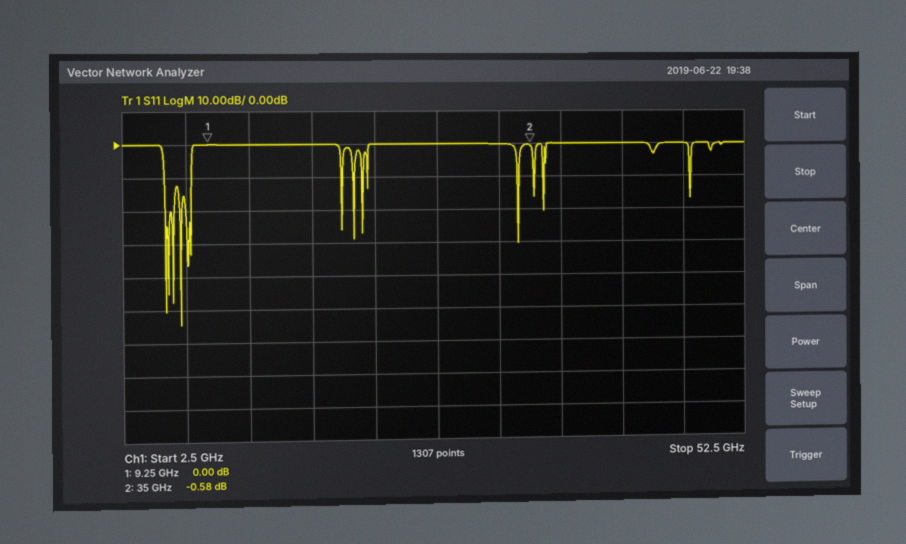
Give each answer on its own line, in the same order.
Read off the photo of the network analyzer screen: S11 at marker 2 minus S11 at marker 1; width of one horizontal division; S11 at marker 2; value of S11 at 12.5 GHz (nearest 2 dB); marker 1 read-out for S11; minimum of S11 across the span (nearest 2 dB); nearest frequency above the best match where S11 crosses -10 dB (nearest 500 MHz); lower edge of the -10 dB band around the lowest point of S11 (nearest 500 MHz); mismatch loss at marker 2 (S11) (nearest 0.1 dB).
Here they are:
-0.58 dB
5 GHz
-0.58 dB
0 dB
0.00 dB
-54 dB
8.0 GHz
6.0 GHz
9.0 dB
